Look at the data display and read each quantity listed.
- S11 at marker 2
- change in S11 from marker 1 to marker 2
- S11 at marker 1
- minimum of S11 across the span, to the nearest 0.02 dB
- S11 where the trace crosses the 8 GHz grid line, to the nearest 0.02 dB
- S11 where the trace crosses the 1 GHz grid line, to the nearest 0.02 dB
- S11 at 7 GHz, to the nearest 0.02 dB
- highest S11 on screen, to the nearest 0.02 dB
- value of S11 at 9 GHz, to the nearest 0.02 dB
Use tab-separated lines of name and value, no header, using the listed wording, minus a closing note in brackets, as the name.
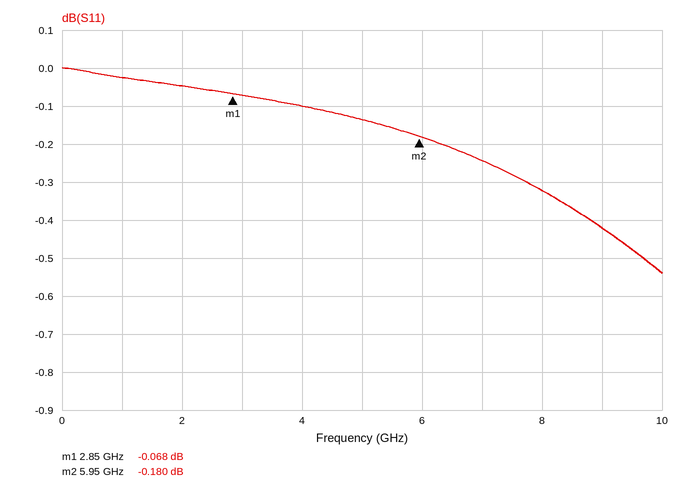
S11 at marker 2	-0.180 dB
change in S11 from marker 1 to marker 2	-0.112 dB
S11 at marker 1	-0.068 dB
minimum of S11 across the span, to the nearest 0.02 dB	-0.54 dB
S11 where the trace crosses the 8 GHz grid line, to the nearest 0.02 dB	-0.32 dB
S11 where the trace crosses the 1 GHz grid line, to the nearest 0.02 dB	-0.02 dB
S11 at 7 GHz, to the nearest 0.02 dB	-0.24 dB
highest S11 on screen, to the nearest 0.02 dB	0.00 dB
value of S11 at 9 GHz, to the nearest 0.02 dB	-0.42 dB
